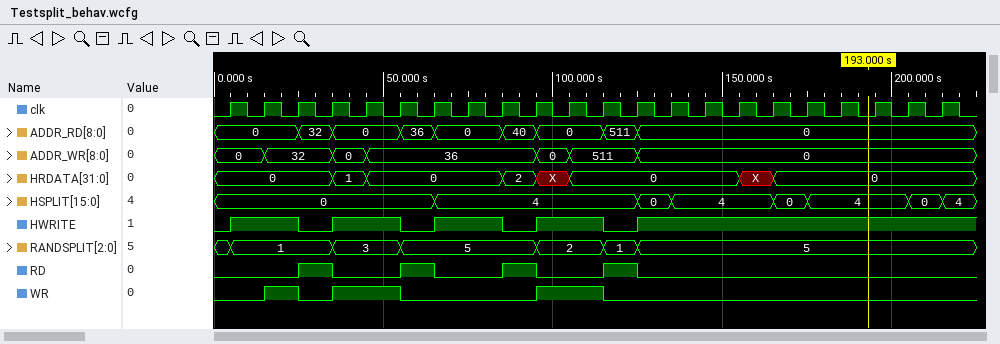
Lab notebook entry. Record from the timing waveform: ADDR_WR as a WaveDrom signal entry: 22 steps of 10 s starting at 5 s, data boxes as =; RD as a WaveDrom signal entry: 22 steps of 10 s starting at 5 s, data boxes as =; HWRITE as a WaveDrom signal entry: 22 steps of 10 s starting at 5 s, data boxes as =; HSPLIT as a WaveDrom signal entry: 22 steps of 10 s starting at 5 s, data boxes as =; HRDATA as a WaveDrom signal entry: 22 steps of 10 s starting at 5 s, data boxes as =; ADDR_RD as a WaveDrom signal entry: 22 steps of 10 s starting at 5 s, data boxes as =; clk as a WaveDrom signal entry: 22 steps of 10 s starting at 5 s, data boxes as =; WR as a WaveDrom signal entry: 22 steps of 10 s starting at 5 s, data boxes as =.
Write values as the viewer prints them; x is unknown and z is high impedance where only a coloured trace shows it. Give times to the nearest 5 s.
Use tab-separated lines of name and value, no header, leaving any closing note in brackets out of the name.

ADDR_WR as a WaveDrom signal entry: 22 steps of 10 s starting at 5 s, data boxes as =	{name: 'ADDR_WR', wave: '==.==....==.=.........', data: '0 32 0 36 0 511 0'}
RD as a WaveDrom signal entry: 22 steps of 10 s starting at 5 s, data boxes as =	{name: 'RD', wave: '0.10.10.10.10.........'}
HWRITE as a WaveDrom signal entry: 22 steps of 10 s starting at 5 s, data boxes as =	{name: 'HWRITE', wave: '1.01.01.01.01.........'}
HSPLIT as a WaveDrom signal entry: 22 steps of 10 s starting at 5 s, data boxes as =	{name: 'HSPLIT', wave: '=.....=.....==..==..==', data: '0 4 0 4 0 4 0 4'}
HRDATA as a WaveDrom signal entry: 22 steps of 10 s starting at 5 s, data boxes as =	{name: 'HRDATA', wave: '=..==...=x=....x=.....', data: '0 1 0 2 0 0'}
ADDR_RD as a WaveDrom signal entry: 22 steps of 10 s starting at 5 s, data boxes as =	{name: 'ADDR_RD', wave: '=.==.==.==.==.........', data: '0 32 0 36 0 40 0 511 0'}
clk as a WaveDrom signal entry: 22 steps of 10 s starting at 5 s, data boxes as =	{name: 'clk', wave: 'p.....................'}
WR as a WaveDrom signal entry: 22 steps of 10 s starting at 5 s, data boxes as =	{name: 'WR', wave: '0101.0...1.0..........'}
